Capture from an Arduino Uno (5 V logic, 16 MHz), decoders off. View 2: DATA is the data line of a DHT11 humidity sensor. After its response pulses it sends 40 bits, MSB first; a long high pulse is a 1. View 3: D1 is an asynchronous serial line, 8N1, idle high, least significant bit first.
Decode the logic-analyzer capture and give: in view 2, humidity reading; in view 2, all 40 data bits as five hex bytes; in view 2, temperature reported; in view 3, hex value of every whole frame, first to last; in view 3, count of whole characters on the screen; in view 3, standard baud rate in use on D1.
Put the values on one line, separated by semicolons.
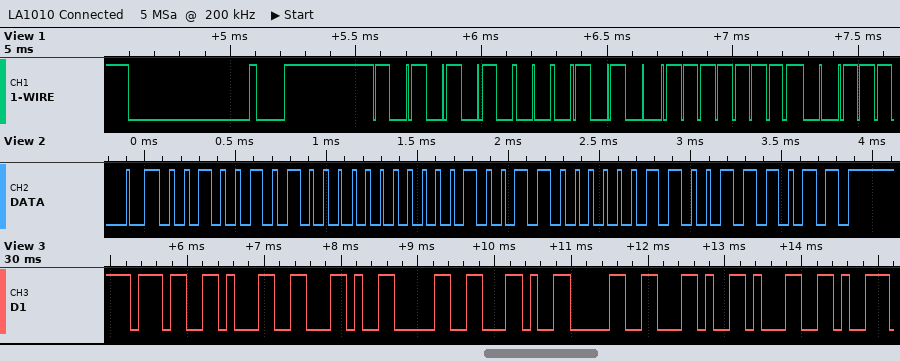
37 %; 25 00 13 03 3B; 19.3 °C; 0x37 0x31 0x2C 0x30 0x2C 0x30 0x2C 0x31; 8; 9600 baud
